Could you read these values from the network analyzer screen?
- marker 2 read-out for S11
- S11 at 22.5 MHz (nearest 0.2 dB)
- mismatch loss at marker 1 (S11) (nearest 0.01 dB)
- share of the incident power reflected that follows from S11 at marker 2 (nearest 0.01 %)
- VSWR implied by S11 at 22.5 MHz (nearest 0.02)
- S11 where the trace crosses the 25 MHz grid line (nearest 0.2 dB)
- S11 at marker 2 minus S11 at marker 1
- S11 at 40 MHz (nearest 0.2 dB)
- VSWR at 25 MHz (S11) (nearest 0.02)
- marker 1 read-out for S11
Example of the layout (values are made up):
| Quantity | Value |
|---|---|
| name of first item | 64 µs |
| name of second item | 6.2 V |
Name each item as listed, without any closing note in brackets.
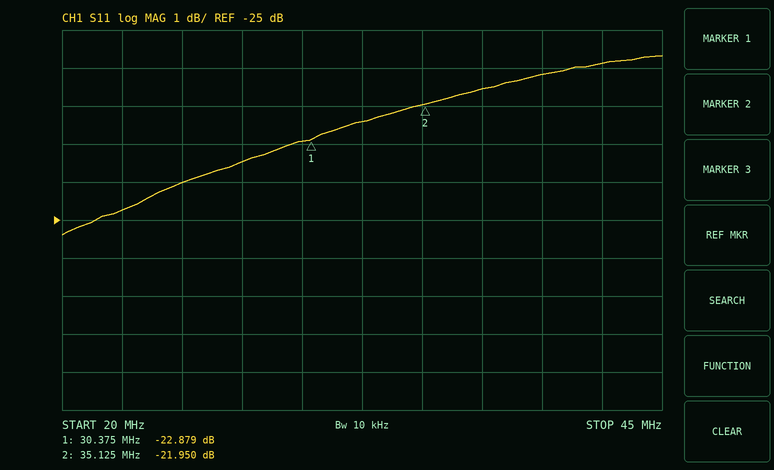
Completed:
| Quantity | Value |
|---|---|
| marker 2 read-out for S11 | -21.950 dB |
| S11 at 22.5 MHz | -24.8 dB |
| mismatch loss at marker 1 (S11) | 0.02 dB |
| share of the incident power reflected that follows from S11 at marker 2 | 0.64 % |
| VSWR implied by S11 at 22.5 MHz | 1.12 |
| S11 where the trace crosses the 25 MHz grid line | -24.0 dB |
| S11 at marker 2 minus S11 at marker 1 | 0.929 dB |
| S11 at 40 MHz | -21.2 dB |
| VSWR at 25 MHz (S11) | 1.14 |
| marker 1 read-out for S11 | -22.879 dB |
